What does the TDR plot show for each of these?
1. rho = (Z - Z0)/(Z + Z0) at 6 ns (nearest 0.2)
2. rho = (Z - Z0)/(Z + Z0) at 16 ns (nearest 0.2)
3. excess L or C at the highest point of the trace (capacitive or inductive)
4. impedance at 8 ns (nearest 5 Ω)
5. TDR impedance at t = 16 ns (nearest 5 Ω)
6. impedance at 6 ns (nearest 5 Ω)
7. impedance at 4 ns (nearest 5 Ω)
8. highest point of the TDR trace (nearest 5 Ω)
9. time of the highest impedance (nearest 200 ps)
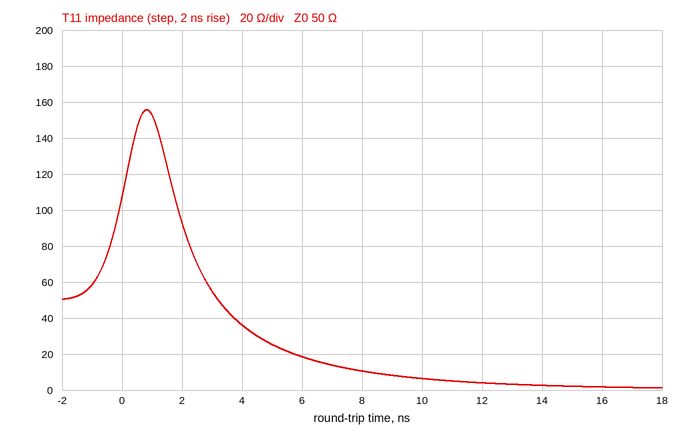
-0.4
-1.0
inductive
10 Ω
0 Ω
20 Ω
35 Ω
155 Ω
800 ps
